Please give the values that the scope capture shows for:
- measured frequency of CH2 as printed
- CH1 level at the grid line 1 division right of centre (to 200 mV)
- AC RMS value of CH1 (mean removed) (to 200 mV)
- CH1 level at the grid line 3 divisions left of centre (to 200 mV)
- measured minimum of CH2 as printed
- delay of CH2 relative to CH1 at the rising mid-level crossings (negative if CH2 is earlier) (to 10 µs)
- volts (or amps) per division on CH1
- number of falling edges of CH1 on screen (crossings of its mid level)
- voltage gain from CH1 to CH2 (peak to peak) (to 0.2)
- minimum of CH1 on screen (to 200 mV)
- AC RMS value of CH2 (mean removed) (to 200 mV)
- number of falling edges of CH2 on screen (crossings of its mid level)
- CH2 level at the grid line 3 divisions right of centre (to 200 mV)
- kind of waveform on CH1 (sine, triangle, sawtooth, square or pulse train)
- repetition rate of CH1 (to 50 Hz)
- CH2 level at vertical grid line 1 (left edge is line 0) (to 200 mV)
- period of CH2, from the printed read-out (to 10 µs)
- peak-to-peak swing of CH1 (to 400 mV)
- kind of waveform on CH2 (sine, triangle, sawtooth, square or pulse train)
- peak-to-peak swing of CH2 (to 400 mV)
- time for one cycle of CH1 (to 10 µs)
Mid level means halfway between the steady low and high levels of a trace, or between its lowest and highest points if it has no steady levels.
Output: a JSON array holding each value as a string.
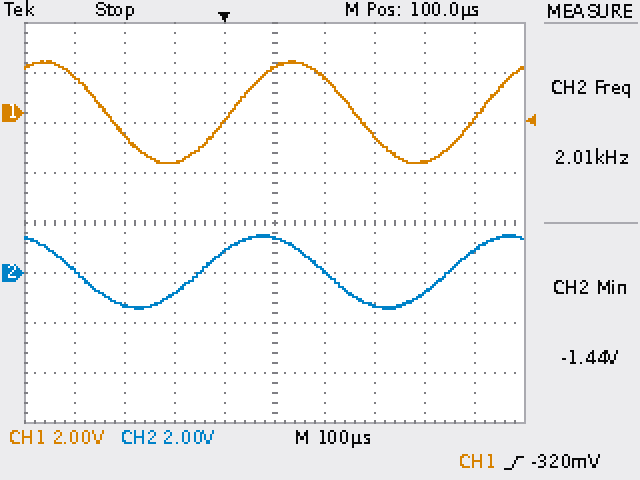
["2.01 kHz", "1.4 V", "1.4 V", "-800 mV", "-1.44 V", "-60 µs", "2 V", "2", "0.8", "-2.0 V", "1.0 V", "2", "-800 mV", "sine", "2.00 kHz", "200 mV", "500 µs", "4.0 V", "sine", "2.8 V", "500 µs"]
